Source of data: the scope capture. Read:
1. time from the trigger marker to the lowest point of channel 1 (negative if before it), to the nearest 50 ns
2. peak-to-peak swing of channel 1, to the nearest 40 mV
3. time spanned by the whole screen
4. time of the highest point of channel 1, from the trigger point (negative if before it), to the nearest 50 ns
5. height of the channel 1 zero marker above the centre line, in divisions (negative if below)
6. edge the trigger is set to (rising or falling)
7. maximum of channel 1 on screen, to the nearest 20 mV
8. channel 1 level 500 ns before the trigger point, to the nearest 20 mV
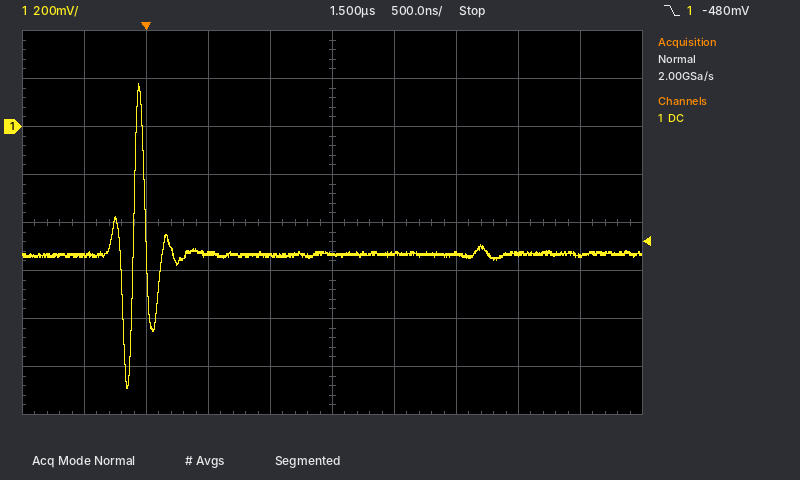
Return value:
-150 ns
1.28 V
5 µs
-50 ns
+2.0 div
falling
180 mV
-540 mV
